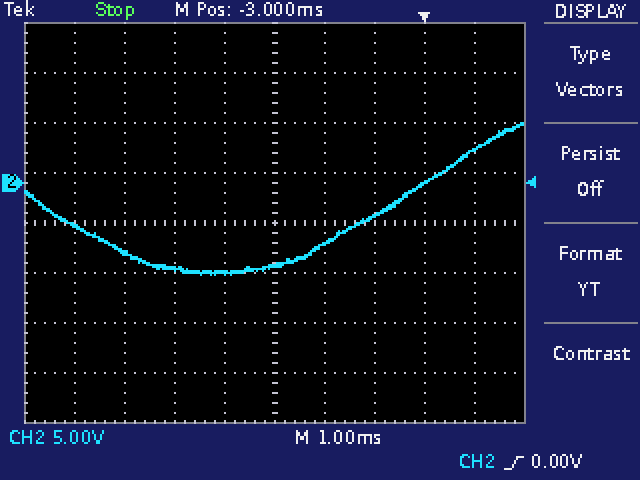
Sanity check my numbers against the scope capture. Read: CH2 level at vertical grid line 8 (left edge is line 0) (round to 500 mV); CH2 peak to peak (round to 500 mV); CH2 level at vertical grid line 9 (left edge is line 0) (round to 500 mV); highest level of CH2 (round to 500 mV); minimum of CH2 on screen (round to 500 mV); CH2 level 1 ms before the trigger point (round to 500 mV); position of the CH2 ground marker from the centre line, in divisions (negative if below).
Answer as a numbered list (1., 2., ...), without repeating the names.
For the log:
1. 0.0 V
2. 15.0 V
3. 3.5 V
4. 6.0 V
5. -9.0 V
6. -3.5 V
7. +0.8 div
